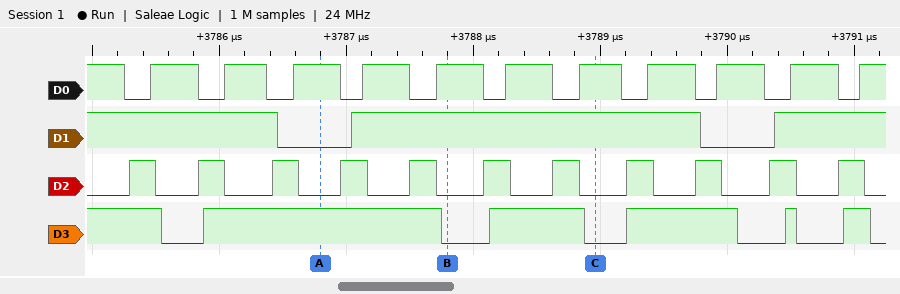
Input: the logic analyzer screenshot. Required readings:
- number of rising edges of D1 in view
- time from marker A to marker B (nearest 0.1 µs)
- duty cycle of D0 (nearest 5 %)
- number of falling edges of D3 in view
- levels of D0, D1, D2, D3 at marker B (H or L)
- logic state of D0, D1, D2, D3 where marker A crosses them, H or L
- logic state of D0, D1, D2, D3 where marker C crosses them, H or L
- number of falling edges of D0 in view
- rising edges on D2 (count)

2
1 µs
65 %
6
D0=H, D1=H, D2=L, D3=L
D0=H, D1=L, D2=L, D3=H
D0=H, D1=H, D2=L, D3=L
11
11
